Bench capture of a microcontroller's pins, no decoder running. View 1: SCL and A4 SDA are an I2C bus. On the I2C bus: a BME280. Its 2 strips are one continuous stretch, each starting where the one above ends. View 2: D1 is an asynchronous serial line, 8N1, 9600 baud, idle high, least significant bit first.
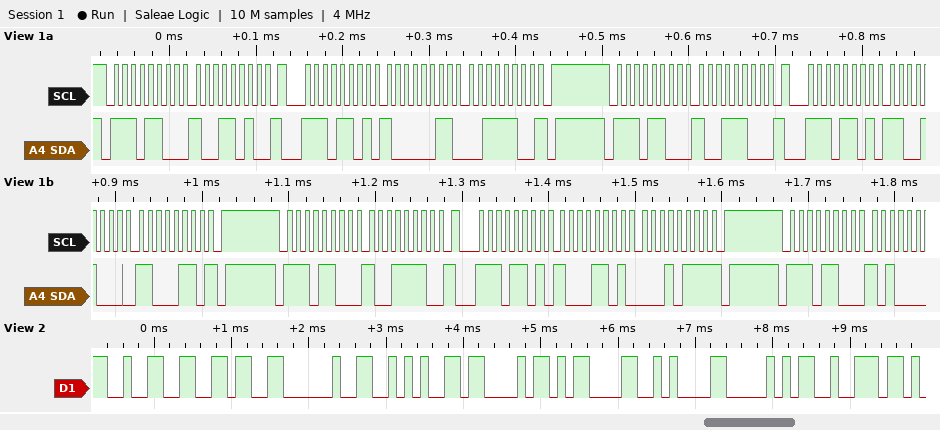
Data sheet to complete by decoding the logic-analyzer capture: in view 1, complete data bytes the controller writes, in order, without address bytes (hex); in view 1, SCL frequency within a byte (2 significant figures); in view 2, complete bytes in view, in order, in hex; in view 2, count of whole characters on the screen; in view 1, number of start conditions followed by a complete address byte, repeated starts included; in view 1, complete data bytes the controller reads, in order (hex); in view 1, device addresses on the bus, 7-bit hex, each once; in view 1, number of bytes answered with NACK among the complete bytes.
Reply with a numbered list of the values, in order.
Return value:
1. 9A 9C 9E
2. 100 kHz
3. 32 36 20 2A 43 0D 0A 50 72
4. 9
5. 7
6. 83 3C C8 C6 8D 17
7. 0x76
8. 3
